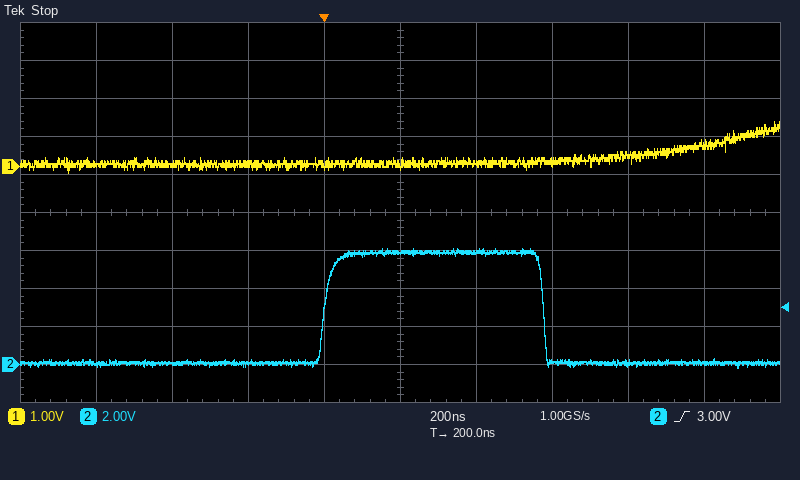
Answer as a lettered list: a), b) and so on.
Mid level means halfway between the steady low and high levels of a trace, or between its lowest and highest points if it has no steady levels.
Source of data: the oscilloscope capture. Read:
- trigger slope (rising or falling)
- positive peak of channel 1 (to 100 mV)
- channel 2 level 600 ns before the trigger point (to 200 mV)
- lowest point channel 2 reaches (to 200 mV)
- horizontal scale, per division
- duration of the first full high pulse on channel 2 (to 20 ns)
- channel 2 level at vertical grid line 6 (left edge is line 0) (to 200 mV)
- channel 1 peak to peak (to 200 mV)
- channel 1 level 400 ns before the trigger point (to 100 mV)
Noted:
a) rising
b) 1.2 V
c) 0.0 V
d) -200 mV
e) 200 ns
f) 580 ns
g) 6.0 V
h) 1.4 V
i) 100 mV
